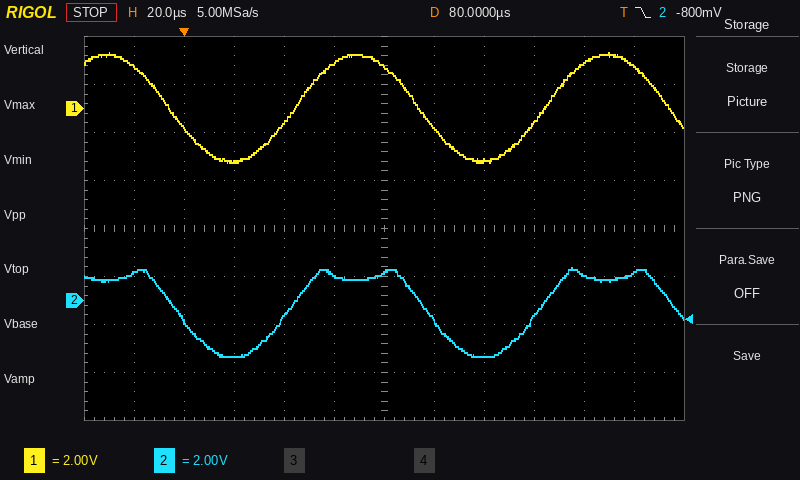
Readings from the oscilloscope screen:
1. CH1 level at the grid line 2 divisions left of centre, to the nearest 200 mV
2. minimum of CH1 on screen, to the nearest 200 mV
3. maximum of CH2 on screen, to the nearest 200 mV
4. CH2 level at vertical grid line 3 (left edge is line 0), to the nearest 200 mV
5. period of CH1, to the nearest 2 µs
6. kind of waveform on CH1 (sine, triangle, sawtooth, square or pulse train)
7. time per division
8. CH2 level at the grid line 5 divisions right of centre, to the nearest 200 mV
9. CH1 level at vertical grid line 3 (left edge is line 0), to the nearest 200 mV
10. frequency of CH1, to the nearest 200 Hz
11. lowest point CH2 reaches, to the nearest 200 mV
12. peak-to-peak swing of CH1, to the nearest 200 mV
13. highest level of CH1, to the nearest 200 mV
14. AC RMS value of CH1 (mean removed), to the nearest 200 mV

-600 mV
-2.2 V
1.4 V
-2.4 V
100 µs
sine
20 µs
1.2 V
-2.2 V
10.0 kHz
-2.4 V
4.6 V
2.4 V
1.6 V
